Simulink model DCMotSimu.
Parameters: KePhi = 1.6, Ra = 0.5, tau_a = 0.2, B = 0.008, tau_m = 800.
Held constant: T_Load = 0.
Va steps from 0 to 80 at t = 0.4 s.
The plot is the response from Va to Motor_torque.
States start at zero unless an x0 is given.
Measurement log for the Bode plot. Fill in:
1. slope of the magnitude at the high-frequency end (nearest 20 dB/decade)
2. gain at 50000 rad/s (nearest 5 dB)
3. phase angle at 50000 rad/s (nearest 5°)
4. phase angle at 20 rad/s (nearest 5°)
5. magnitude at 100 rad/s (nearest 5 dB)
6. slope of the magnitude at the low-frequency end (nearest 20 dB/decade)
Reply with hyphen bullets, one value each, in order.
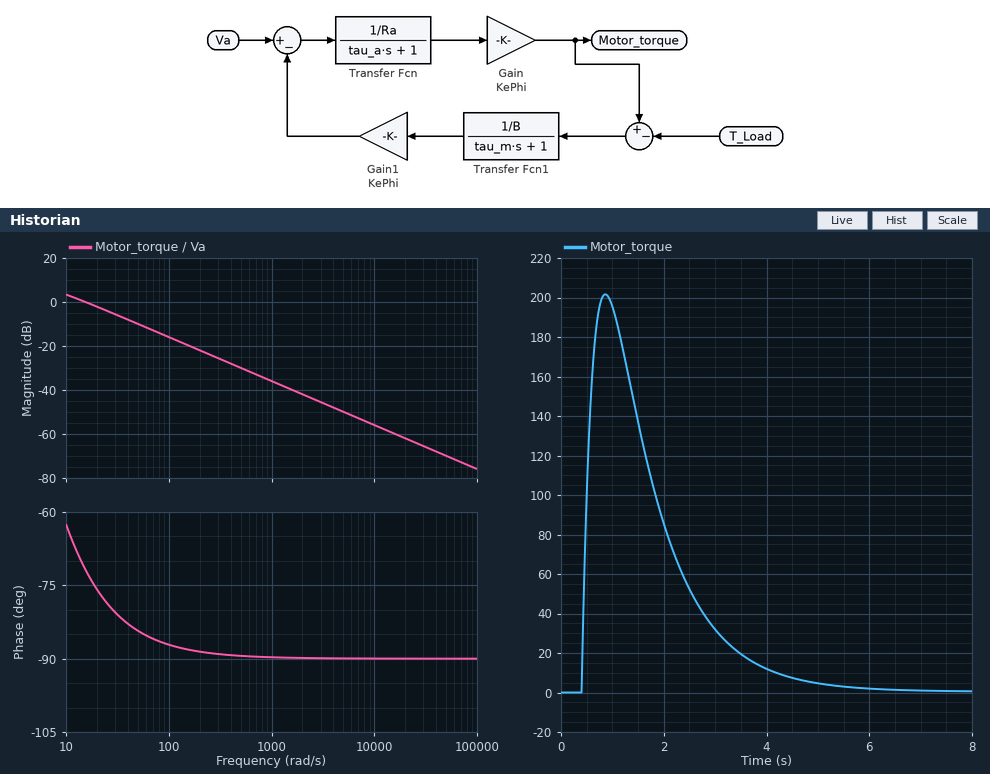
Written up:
- -20 dB/decade
- -70 dB
- -90°
- -75°
- -15 dB
- -20 dB/decade
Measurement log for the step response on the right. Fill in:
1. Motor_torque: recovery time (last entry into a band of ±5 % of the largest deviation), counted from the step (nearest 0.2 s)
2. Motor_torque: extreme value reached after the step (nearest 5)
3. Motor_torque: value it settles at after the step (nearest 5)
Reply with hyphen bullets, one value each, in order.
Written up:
- 3.8 s
- 200
- 0
